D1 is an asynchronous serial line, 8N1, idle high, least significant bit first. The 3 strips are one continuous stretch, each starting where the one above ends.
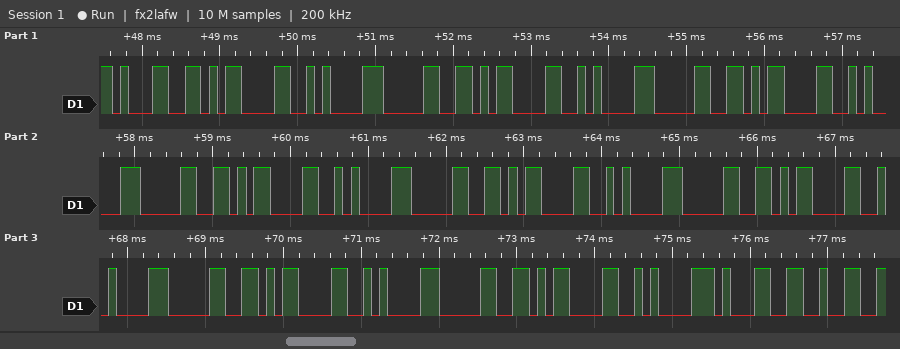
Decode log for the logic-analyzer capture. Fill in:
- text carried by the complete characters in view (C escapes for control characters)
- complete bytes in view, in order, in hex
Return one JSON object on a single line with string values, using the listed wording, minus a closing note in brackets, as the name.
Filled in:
{"text carried by the complete characters in view": "\"1\\r\\n0\\r\\n0\\r\\n0\\r\\n0\\r\\n0\\r\\n0\\r\\n0\\r\\n12\"", "complete bytes in view, in order, in hex": "0x31 0x0D 0x0A 0x30 0x0D 0x0A 0x30 0x0D 0x0A 0x30 0x0D 0x0A 0x30 0x0D 0x0A 0x30 0x0D 0x0A 0x30 0x0D 0x0A 0x30 0x0D 0x0A 0x31 0x32"}
